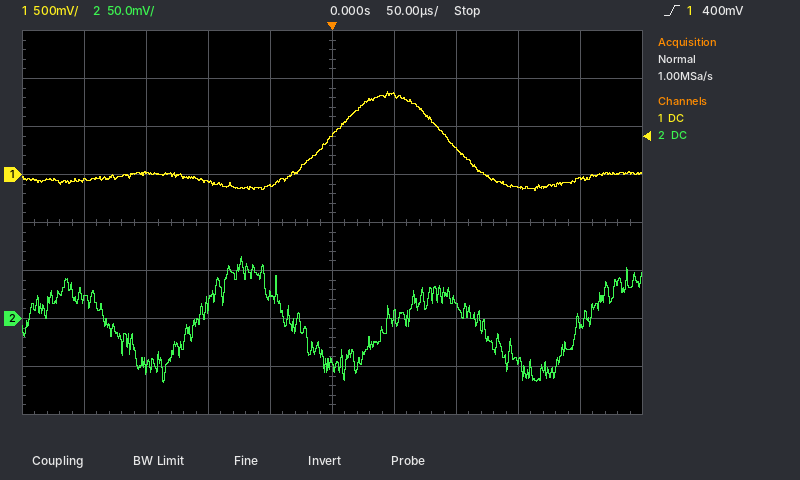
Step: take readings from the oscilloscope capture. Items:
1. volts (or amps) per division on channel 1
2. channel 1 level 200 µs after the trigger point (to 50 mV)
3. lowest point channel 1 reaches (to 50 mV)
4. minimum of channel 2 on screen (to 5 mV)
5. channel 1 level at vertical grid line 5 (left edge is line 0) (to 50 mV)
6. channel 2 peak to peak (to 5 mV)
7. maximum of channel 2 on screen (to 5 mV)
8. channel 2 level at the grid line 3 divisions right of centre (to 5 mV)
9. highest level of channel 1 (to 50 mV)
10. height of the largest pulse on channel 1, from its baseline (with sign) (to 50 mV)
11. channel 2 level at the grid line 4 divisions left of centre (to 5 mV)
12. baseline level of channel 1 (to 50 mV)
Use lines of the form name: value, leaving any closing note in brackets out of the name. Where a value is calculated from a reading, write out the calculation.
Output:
volts (or amps) per division on channel 1: 500 mV
channel 1 level 200 µs after the trigger point: -50 mV
lowest point channel 1 reaches: -150 mV
minimum of channel 2 on screen: -65 mV
channel 1 level at vertical grid line 5 (left edge is line 0): 400 mV
channel 2 peak to peak: 65 mV − (-65 mV) = 130 mV
maximum of channel 2 on screen: 65 mV
channel 2 level at the grid line 3 divisions right of centre: -45 mV
highest level of channel 1: 850 mV
height of the largest pulse on channel 1, from its baseline (with sign): 850 mV − (-50 mV) = +900 mV
channel 2 level at the grid line 4 divisions left of centre: 20 mV
baseline level of channel 1: -50 mV
